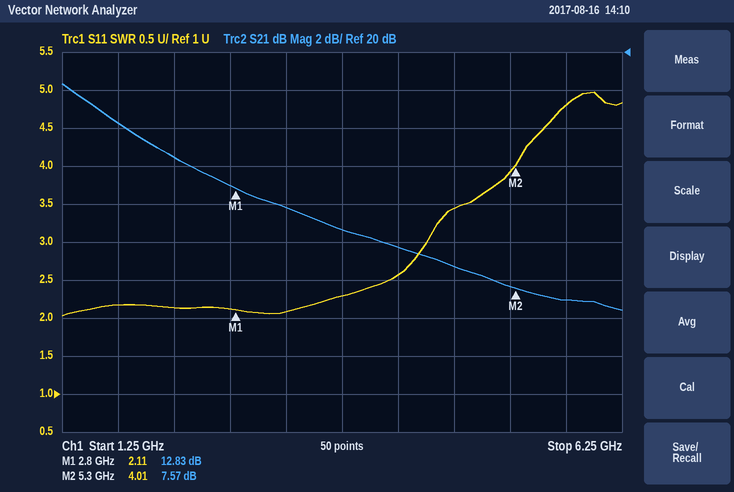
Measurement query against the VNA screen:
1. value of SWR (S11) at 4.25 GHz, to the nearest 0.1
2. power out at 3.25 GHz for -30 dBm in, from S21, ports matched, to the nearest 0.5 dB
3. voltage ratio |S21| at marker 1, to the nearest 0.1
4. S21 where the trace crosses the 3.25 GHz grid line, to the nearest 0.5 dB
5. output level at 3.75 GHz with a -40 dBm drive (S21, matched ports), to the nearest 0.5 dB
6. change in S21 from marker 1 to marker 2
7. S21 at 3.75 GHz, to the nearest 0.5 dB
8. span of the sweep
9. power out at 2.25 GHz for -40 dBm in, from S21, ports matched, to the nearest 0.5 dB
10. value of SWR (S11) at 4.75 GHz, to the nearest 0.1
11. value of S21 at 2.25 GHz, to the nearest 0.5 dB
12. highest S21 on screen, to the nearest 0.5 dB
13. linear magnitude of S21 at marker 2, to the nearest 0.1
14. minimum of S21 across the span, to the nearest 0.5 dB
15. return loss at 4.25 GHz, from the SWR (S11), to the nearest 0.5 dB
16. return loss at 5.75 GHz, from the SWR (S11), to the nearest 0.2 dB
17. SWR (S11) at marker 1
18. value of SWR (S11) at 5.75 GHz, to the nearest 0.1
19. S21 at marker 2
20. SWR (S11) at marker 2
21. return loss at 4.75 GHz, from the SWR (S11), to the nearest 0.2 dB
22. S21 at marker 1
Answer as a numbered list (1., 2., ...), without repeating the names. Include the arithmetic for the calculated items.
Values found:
1. 2.6
2. -30 dBm + (12.0 dB) = -18.0 dBm
3. 10^(12.83/20) ≈ 4.4
4. 12.0 dB
5. -40 dBm + (10.5 dB) = -29.5 dBm
6. 7.57 − (12.83) = -5.26 dB
7. 10.5 dB
8. 5 GHz
9. -40 dBm + (14.5 dB) = -25.5 dBm
10. 3.4
11. 14.5 dB
12. 18.5 dB
13. 10^(7.57/20) ≈ 2.4
14. 6.5 dB
15. −20 log10((2.6 − 1)/(2.6 + 1)) ≈ 7.0 dB
16. −20 log10((4.8 − 1)/(4.8 + 1)) ≈ 3.67 dB, so 3.6 dB to the nearest 0.2 dB
17. 2.11
18. 4.8
19. 7.57 dB
20. 4.01
21. −20 log10((3.4 − 1)/(3.4 + 1)) ≈ 5.26 dB, so 5.2 dB to the nearest 0.2 dB
22. 12.83 dB
